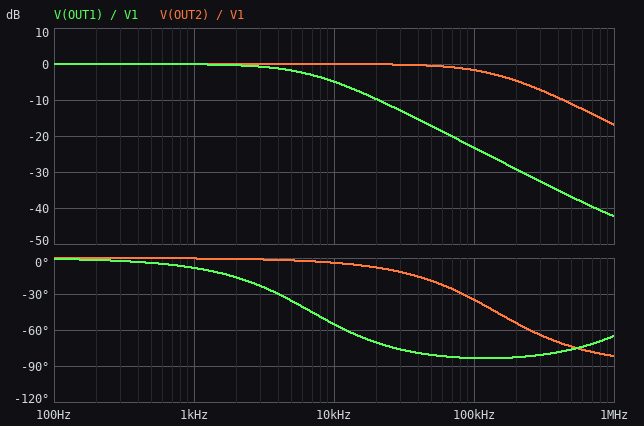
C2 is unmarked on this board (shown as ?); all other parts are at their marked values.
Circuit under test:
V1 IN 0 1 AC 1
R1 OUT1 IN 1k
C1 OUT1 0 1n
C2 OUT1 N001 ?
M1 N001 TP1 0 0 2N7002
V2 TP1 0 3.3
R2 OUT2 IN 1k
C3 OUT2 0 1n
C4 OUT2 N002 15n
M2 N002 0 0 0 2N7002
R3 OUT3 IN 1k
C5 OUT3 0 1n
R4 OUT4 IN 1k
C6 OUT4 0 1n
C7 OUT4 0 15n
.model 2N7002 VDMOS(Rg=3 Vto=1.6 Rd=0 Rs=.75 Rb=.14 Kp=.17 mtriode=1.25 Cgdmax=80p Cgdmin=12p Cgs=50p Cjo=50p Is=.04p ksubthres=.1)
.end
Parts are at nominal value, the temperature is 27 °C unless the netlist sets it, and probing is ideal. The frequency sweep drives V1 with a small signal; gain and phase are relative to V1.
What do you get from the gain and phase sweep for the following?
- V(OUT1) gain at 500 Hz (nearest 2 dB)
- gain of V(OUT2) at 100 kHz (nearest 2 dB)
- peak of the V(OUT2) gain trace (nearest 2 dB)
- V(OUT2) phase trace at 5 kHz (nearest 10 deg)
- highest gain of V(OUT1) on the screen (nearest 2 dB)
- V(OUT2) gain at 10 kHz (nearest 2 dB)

0 dB
-2 dB
0 dB
0 deg
0 dB
0 dB
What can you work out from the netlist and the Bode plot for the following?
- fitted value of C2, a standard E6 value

22 nF
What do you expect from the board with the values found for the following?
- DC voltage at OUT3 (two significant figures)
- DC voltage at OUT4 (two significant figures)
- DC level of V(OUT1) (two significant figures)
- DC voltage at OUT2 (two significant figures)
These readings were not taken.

1.0 V
1.0 V
1.0 V
1.0 V
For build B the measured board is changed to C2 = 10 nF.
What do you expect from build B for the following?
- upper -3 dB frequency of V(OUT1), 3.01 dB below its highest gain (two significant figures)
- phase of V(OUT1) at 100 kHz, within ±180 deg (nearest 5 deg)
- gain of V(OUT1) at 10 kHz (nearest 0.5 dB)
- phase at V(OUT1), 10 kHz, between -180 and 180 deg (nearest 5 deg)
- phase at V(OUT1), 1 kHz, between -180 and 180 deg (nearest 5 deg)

14 kHz
-80 deg
-1.5 dB
-35 deg
-5 deg
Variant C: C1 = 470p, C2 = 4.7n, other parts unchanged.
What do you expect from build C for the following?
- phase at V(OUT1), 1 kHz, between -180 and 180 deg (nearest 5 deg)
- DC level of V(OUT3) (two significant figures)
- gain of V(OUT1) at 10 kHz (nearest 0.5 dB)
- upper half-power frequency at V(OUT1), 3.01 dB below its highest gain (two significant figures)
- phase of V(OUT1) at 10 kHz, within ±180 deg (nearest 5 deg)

0 deg
1.0 V
-0.5 dB
31 kHz
-20 deg
